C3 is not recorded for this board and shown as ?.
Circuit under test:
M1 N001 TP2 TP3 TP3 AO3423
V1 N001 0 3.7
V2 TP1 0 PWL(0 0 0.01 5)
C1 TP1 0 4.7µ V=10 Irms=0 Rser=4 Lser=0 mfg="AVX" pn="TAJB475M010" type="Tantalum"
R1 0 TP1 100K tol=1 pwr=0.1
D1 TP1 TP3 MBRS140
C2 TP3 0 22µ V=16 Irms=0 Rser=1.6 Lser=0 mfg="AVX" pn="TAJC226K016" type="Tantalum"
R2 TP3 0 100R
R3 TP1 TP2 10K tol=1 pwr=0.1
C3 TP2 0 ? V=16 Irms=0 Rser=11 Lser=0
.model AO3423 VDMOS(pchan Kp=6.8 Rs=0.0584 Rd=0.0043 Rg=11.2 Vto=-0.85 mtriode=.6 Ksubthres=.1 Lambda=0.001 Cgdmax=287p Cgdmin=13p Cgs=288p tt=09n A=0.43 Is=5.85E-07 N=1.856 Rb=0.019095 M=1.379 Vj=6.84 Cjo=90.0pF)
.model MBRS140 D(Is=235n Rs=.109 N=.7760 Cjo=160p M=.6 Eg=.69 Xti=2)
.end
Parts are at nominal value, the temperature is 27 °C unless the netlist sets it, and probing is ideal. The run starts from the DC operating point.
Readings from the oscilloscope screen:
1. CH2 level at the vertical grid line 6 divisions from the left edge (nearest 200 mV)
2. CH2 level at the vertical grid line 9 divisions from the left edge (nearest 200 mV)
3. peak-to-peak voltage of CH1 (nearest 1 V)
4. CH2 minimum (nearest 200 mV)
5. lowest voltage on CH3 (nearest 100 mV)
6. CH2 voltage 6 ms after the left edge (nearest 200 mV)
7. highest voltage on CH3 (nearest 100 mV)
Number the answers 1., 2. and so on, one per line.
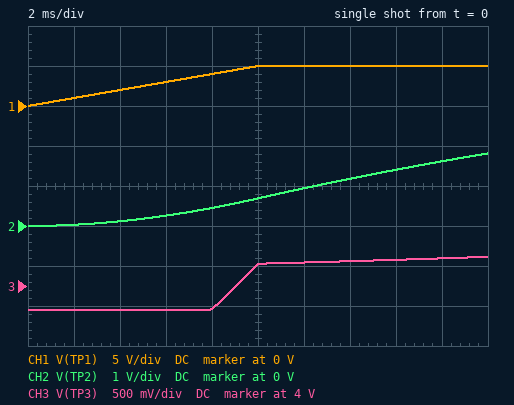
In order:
1. 1.0 V
2. 1.6 V
3. 5 V
4. 0 V
5. 3.7 V
6. 200 mV
7. 4.4 V
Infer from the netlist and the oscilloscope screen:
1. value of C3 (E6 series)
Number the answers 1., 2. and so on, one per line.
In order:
1. 3.3 µF
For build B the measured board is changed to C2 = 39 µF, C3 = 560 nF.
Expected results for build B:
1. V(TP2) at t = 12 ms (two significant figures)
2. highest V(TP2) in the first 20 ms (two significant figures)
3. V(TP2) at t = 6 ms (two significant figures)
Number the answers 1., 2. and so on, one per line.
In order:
1. 3.4 V
2. 4.6 V
3. 1.2 V
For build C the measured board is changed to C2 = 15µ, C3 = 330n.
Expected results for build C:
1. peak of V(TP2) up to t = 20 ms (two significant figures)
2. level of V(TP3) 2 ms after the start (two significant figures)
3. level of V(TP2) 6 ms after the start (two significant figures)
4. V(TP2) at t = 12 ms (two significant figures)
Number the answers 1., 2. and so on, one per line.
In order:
1. 4.9 V
2. 3.7 V
3. 1.6 V
4. 4.1 V
